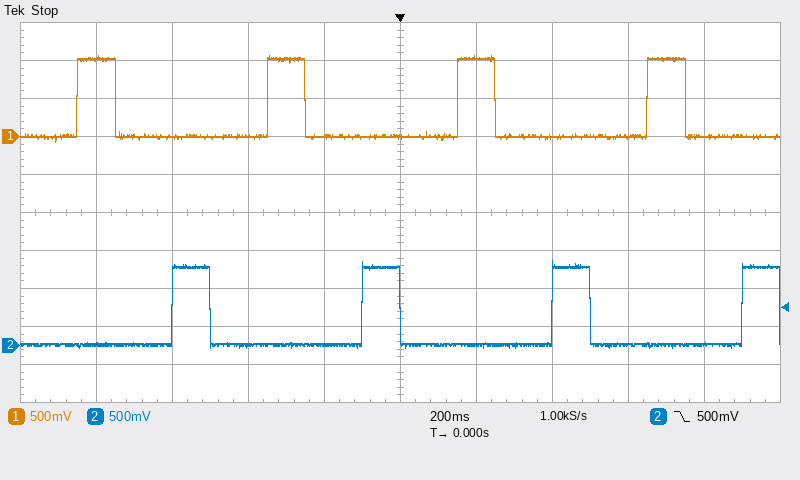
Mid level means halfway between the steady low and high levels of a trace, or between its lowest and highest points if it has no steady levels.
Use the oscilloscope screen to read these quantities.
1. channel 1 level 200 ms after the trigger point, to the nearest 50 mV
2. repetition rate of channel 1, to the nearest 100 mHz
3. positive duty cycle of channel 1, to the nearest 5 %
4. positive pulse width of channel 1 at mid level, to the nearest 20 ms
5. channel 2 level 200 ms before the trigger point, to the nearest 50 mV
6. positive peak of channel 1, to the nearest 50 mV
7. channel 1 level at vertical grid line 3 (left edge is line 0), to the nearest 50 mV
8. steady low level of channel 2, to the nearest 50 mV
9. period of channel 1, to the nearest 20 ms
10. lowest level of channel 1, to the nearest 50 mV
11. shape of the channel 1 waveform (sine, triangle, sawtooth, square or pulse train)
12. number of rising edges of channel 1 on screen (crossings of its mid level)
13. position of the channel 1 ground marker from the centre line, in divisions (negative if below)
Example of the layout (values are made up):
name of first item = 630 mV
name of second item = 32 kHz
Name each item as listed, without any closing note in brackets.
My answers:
channel 1 level 200 ms after the trigger point, to the nearest 50 mV = 1.05 V
repetition rate of channel 1, to the nearest 100 mHz = 2.0 Hz
positive duty cycle of channel 1, to the nearest 5 % = 20 %
positive pulse width of channel 1 at mid level, to the nearest 20 ms = 100 ms
channel 2 level 200 ms before the trigger point, to the nearest 50 mV = 0 mV
positive peak of channel 1, to the nearest 50 mV = 1.05 V
channel 1 level at vertical grid line 3 (left edge is line 0), to the nearest 50 mV = 0 mV
steady low level of channel 2, to the nearest 50 mV = 0 mV
period of channel 1, to the nearest 20 ms = 500 ms
lowest level of channel 1, to the nearest 50 mV = -50 mV
shape of the channel 1 waveform = pulse train
number of rising edges of channel 1 on screen = 4
position of the channel 1 ground marker from the centre line, in divisions = +2.0 div
